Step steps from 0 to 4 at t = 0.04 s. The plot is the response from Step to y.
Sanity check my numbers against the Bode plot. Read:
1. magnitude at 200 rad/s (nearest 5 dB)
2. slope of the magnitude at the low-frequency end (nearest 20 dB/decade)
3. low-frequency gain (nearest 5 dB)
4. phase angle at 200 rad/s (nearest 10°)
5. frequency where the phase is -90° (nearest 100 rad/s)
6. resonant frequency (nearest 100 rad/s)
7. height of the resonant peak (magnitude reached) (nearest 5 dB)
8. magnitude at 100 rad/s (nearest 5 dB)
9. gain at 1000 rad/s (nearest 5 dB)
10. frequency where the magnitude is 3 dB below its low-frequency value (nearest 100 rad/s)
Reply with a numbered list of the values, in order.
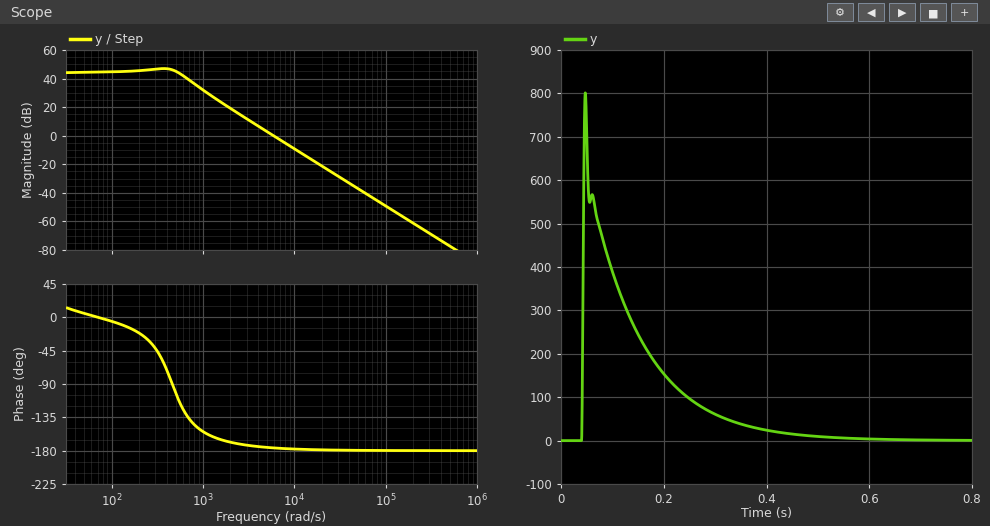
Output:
1. 45 dB
2. 0 dB/decade
3. 45 dB
4. -20°
5. 500 rad/s
6. 400 rad/s
7. 45 dB
8. 45 dB
9. 30 dB
10. 600 rad/s
